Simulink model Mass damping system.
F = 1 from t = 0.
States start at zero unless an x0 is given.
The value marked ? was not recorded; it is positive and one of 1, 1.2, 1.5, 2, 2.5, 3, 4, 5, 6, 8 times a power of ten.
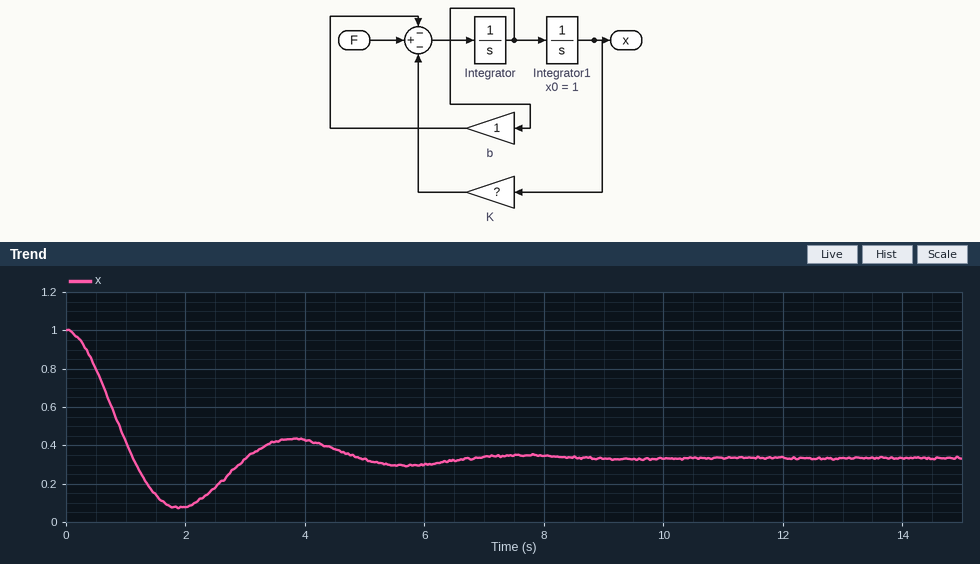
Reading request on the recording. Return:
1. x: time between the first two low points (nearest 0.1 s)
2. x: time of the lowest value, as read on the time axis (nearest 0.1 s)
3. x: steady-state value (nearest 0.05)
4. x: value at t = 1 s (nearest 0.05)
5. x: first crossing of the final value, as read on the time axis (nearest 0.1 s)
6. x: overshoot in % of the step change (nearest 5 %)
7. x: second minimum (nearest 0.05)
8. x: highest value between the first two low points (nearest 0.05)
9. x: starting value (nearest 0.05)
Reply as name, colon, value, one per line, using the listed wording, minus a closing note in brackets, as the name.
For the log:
x: time between the first two low points: 3.8 s
x: time of the lowest value, as read on the time axis: 1.9 s
x: steady-state value: 0.35
x: value at t = 1 s: 0.40
x: first crossing of the final value, as read on the time axis: 1.1 s
x: overshoot in % of the step change: 40 %
x: second minimum: 0.30
x: highest value between the first two low points: 0.45
x: starting value: 1.00
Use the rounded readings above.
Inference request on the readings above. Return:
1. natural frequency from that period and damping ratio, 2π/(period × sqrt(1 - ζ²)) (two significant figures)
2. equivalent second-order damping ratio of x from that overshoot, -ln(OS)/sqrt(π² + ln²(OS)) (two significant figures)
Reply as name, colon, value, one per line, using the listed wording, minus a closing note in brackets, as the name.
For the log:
natural frequency from that period and damping ratio, 2π/(period × sqrt(1 - ζ²)): 1.7 rad/s
equivalent second-order damping ratio of x from that overshoot, -ln(OS)/sqrt(π² + ln²(OS)): 0.28
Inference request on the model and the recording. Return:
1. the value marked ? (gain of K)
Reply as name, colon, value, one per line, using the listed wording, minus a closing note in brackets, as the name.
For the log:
the value marked ?: 3
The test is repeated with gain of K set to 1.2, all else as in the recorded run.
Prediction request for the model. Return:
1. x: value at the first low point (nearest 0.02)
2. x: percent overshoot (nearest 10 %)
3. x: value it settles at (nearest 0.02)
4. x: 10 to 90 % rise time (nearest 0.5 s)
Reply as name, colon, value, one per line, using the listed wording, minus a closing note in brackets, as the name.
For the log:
x: value at the first low point: 0.80
x: percent overshoot: 20 %
x: value it settles at: 0.84
x: 10 to 90 % rise time: 1.5 s
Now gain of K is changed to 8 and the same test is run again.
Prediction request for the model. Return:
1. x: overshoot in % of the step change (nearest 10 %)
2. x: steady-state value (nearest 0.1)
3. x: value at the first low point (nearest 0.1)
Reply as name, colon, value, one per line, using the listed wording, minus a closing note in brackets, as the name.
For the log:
x: overshoot in % of the step change: 60 %
x: steady-state value: 0.1
x: value at the first low point: -0.4
